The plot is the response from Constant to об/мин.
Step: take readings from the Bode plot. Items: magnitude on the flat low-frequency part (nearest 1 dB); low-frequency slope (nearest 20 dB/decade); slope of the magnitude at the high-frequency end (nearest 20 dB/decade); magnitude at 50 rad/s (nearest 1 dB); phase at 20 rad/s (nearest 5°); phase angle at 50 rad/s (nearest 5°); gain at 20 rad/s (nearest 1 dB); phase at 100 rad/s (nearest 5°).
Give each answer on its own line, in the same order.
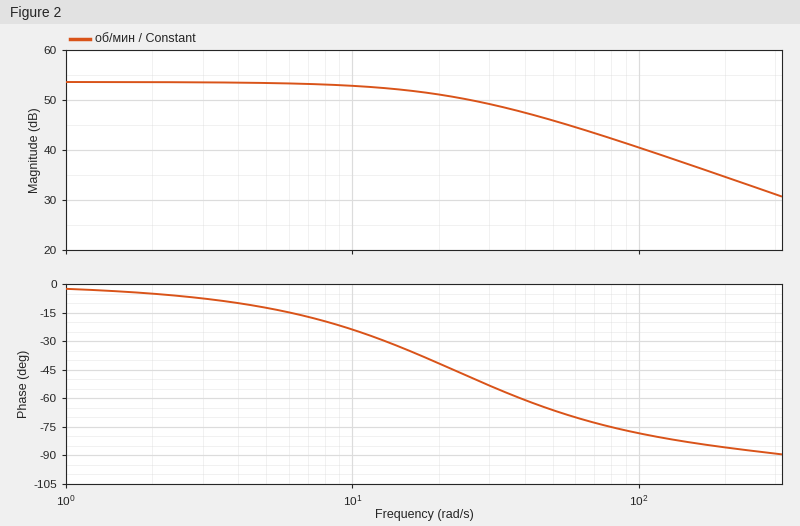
54 dB
0 dB/decade
-20 dB/decade
46 dB
-40°
-65°
51 dB
-80°
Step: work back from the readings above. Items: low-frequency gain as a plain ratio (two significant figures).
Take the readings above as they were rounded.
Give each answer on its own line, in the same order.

500
